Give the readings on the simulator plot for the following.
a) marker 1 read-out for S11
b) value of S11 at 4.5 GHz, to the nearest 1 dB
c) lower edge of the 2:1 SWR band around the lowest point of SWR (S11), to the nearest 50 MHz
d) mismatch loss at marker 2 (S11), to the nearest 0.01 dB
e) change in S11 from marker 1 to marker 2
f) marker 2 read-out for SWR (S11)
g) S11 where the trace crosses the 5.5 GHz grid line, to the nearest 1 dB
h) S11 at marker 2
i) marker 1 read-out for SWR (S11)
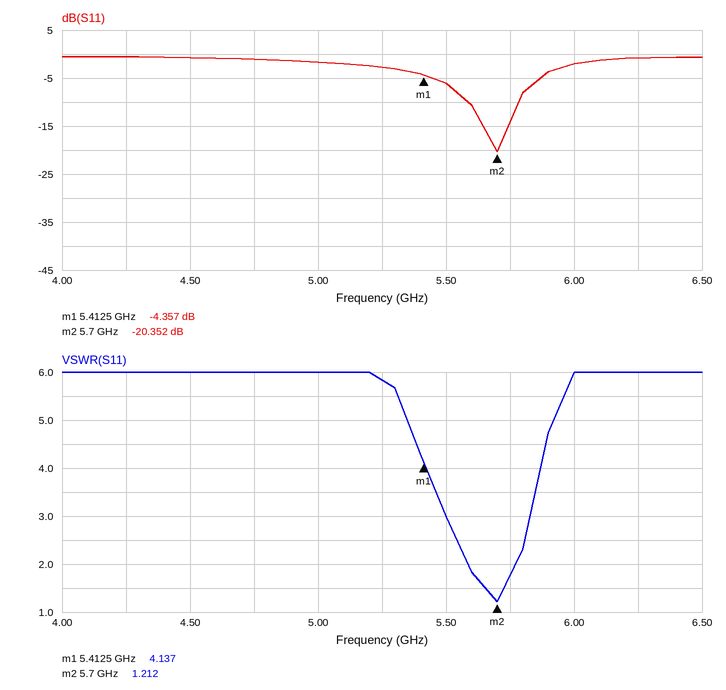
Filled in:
-4.357 dB
-1 dB
5.60 GHz
0.04 dB
-15.995 dB
1.212
-6 dB
-20.352 dB
4.137
